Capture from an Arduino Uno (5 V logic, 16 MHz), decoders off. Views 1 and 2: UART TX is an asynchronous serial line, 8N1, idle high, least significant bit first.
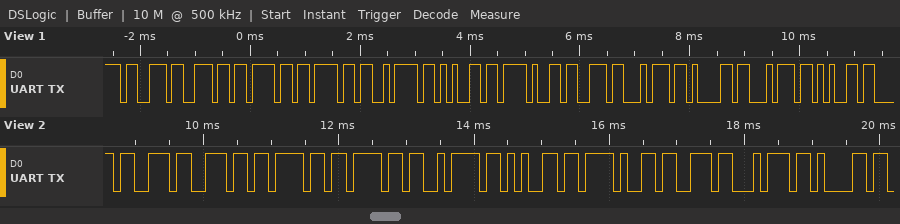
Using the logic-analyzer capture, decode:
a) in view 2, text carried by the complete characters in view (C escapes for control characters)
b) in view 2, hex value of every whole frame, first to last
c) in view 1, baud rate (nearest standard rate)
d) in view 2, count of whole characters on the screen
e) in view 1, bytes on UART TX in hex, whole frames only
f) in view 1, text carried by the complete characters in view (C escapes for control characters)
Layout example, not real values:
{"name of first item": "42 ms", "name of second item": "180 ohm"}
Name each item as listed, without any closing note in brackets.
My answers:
{"in view 2, text carried by the complete characters in view": "\"snooze/sta\"", "in view 2, hex value of every whole frame, first to last": "73 6E 6F 6F 7A 65 2F 73 74 61", "in view 1, baud rate": "9600 baud", "in view 2, count of whole characters on the screen": "10", "in view 1, bytes on UART TX in hex, whole frames only": "73 6E 6F 6F 7A 65 2F 73 74 61 74 65", "in view 1, text carried by the complete characters in view": "\"snooze/state\""}
